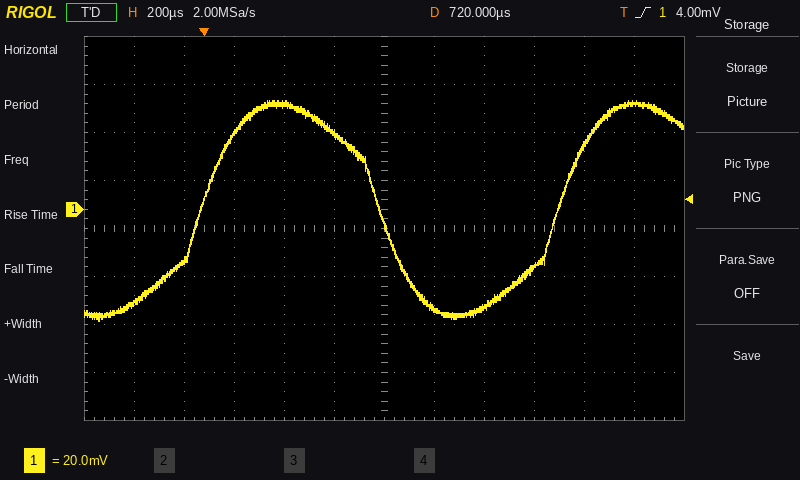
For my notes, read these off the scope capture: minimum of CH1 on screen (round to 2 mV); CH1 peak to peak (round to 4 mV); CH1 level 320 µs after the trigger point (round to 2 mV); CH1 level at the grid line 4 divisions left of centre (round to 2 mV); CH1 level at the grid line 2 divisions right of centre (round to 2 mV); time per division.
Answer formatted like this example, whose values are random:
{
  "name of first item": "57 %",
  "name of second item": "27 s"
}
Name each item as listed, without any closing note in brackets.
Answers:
{
  "minimum of CH1 on screen": "-46 mV",
  "CH1 peak to peak": "92 mV",
  "CH1 level 320 µs after the trigger point": "44 mV",
  "CH1 level at the grid line 4 divisions left of centre": "-22 mV",
  "CH1 level at the grid line 2 divisions right of centre": "-42 mV",
  "time per division": "200 µs"
}
